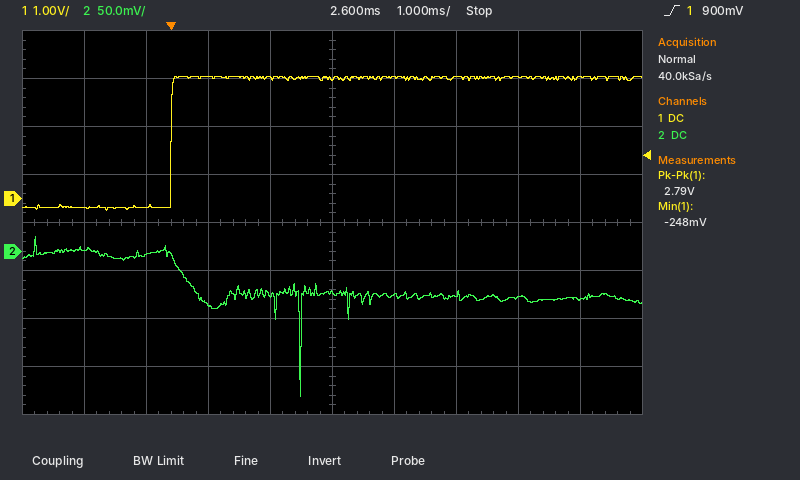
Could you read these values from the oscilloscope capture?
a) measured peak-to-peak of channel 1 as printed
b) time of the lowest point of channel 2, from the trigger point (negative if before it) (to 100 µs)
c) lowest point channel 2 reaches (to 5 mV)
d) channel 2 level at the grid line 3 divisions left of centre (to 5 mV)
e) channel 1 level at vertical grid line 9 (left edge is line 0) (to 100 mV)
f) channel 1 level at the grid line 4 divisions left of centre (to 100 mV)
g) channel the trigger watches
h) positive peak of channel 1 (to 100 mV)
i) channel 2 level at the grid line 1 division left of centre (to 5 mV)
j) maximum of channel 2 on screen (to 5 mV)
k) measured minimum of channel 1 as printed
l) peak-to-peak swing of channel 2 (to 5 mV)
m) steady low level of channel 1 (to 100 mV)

2.79 V
+2.1 ms
-150 mV
-5 mV
2.5 V
-200 mV
channel 1
2.5 V
-45 mV
15 mV
-248 mV
165 mV
-200 mV
